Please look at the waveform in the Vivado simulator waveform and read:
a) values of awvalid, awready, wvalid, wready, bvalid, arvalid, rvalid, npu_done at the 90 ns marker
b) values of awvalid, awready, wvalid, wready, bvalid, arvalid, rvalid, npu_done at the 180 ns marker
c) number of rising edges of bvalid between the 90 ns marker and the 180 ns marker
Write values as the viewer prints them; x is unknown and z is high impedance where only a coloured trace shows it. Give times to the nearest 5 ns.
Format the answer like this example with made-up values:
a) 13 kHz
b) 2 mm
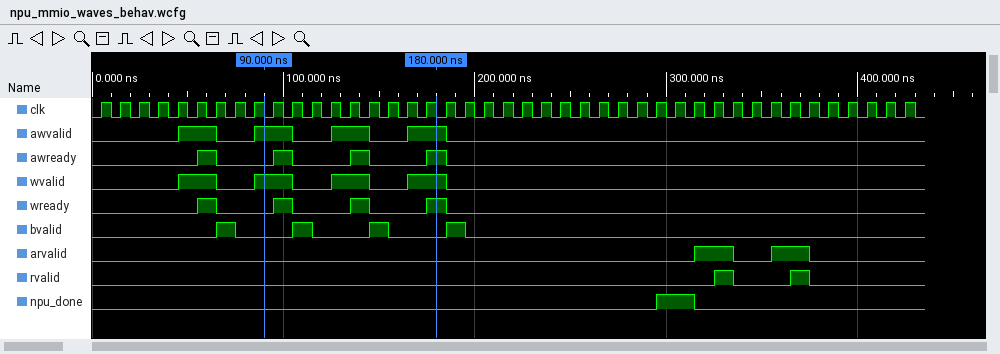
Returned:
a) awvalid=1, awready=0, wvalid=1, wready=0, bvalid=0, arvalid=0, rvalid=0, npu_done=0
b) awvalid=1, awready=1, wvalid=1, wready=1, bvalid=0, arvalid=0, rvalid=0, npu_done=0
c) 2
